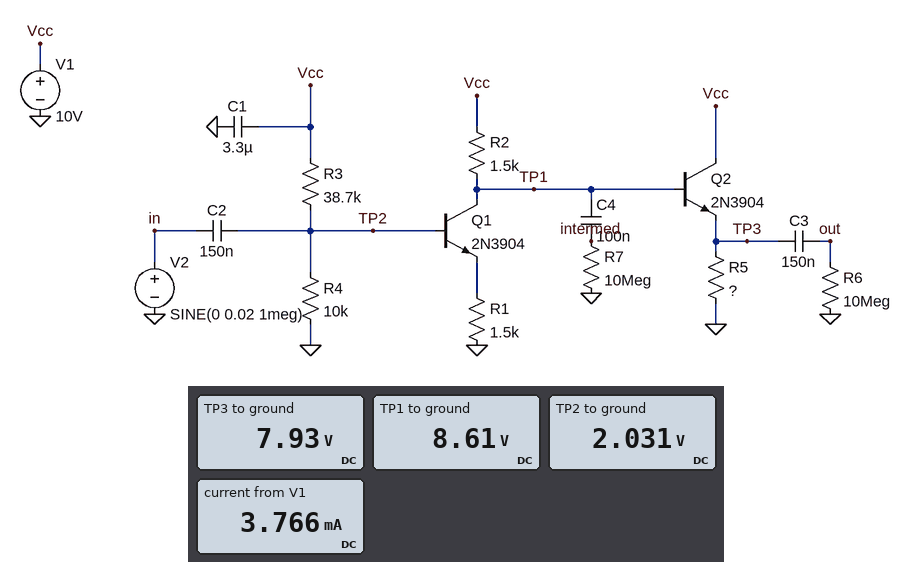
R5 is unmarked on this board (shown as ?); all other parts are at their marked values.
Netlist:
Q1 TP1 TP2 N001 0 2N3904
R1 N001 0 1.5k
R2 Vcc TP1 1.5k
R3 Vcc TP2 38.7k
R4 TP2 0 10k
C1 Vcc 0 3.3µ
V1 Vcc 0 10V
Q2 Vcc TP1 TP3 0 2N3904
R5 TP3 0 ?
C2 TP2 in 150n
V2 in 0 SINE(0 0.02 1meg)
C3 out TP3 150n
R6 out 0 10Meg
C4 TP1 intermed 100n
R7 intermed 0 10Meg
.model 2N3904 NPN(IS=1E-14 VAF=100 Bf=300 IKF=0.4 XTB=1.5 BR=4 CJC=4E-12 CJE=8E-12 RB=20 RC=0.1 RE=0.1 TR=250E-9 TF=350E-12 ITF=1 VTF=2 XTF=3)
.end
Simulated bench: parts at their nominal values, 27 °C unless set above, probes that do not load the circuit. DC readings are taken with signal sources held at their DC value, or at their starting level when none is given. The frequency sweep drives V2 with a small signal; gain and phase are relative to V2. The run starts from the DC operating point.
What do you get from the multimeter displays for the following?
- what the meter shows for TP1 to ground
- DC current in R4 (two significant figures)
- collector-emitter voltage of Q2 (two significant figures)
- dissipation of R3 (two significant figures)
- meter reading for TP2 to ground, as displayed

8.61 V
200 µA
2.1 V
1.6 mW
2.031 V
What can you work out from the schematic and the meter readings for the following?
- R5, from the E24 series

3 kΩ
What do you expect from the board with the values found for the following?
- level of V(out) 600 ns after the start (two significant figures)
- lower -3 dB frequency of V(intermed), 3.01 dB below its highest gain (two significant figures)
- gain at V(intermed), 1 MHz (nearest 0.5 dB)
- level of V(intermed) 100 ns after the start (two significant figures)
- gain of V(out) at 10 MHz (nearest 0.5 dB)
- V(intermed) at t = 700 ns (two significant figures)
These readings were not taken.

10 mV
140 Hz
0 dB
-10 mV
-1.0 dB
18 mV
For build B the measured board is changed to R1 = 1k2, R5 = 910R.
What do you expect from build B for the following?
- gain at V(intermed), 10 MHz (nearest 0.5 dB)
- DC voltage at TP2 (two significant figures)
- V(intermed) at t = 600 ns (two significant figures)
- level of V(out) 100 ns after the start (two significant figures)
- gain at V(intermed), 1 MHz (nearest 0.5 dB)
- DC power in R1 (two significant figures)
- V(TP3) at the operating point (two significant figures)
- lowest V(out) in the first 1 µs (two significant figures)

1.0 dB
2.0 V
13 mV
-13 mV
1.5 dB
1.6 mW
7.5 V
-24 mV
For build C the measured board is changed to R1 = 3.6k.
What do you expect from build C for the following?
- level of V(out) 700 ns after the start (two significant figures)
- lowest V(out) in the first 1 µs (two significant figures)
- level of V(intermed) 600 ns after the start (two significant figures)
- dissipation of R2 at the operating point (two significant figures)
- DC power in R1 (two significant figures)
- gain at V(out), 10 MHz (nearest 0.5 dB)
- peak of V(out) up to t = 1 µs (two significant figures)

7.4 mV
-8.1 mV
4.1 mV
240 µW
560 µW
-8.0 dB
8.1 mV
